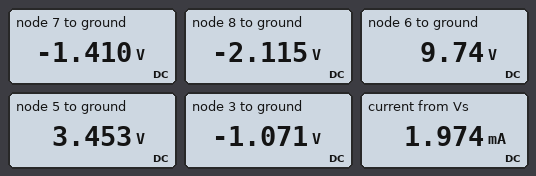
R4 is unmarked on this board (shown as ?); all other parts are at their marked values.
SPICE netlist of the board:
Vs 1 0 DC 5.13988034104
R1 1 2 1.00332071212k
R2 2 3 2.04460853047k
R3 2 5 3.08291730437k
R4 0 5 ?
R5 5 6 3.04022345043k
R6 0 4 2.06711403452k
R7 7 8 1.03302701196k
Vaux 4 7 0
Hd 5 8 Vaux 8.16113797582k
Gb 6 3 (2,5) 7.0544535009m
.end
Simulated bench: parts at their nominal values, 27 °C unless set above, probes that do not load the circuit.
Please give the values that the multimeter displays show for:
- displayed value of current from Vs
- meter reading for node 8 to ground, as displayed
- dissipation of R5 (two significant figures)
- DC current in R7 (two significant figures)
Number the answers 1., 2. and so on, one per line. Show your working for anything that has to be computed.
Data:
1. 1.974 mA
2. -2.115 V
3. (9.74 V - 3.453 V)^2 / 3.04 kΩ = 13 mW
4. (-1.41 V - (-2.115 V)) / 1.033 kΩ = 680 µA
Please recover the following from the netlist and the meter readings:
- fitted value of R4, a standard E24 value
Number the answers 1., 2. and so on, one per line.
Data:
1. 1.3 kΩ
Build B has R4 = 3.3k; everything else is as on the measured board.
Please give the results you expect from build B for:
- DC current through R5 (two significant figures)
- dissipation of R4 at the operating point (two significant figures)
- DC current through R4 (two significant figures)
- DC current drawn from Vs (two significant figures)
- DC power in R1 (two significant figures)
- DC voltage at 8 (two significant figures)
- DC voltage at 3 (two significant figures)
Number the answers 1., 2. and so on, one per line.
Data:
1. 520 µA
2. 6.7 mW
3. 1.4 mA
4. 500 µA
5. 250 µW
6. -2.9 V
7. 3.6 V
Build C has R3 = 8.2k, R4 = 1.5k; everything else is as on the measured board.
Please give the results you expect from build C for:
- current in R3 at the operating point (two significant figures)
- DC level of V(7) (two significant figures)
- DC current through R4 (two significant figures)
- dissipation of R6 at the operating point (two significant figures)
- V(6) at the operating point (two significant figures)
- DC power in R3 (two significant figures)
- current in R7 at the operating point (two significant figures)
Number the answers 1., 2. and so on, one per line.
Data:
1. 30 µA
2. -1.5 V
3. 2.4 mA
4. 1.1 mW
5. 9.0 V
6. 7.5 µW
7. 720 µA
